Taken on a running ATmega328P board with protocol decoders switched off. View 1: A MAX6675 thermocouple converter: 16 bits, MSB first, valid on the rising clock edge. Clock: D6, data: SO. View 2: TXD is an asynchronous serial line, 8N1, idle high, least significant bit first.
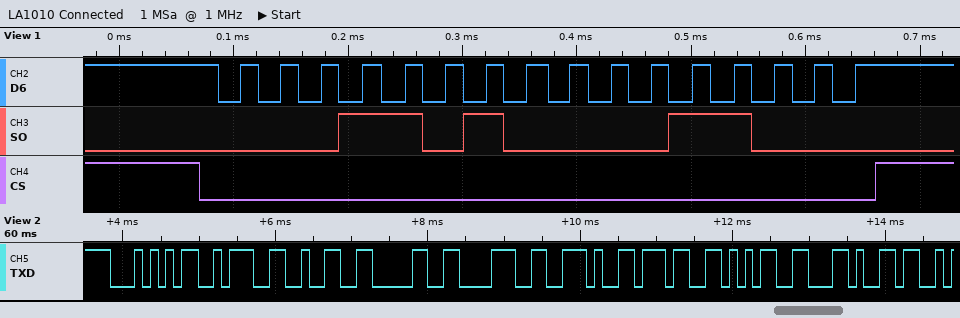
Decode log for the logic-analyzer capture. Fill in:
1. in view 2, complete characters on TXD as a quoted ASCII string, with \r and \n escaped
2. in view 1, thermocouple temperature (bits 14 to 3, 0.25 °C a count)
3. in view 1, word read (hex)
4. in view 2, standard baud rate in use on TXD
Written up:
"T:208.75,"
208.75 °C
0x1A18
9600 baud
